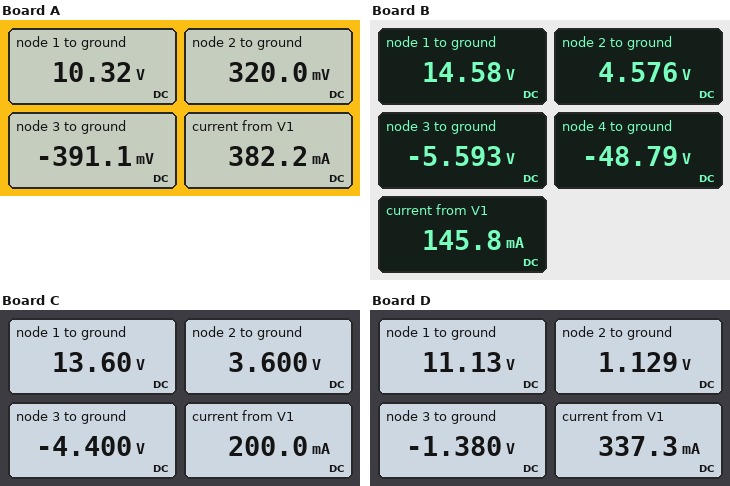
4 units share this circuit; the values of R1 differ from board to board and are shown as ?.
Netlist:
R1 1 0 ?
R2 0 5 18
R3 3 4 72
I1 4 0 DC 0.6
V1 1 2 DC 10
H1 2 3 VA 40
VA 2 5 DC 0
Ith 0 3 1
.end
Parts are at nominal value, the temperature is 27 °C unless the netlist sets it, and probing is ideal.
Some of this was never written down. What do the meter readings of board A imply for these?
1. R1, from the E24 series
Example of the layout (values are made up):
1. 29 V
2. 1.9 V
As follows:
1. 27 Ω
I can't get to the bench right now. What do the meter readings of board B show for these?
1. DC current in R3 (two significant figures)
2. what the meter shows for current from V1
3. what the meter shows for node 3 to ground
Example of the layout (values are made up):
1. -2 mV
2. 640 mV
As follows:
1. 600 mA
2. 145.8 mA
3. -5.593 V
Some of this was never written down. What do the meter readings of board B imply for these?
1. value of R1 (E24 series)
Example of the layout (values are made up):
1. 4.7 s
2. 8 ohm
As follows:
1. 100 Ω
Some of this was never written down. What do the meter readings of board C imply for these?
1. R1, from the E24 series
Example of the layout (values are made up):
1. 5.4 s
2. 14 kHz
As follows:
1. 68 Ω
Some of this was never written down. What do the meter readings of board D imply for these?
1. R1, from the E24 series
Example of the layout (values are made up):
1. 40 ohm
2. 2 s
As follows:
1. 33 Ω
